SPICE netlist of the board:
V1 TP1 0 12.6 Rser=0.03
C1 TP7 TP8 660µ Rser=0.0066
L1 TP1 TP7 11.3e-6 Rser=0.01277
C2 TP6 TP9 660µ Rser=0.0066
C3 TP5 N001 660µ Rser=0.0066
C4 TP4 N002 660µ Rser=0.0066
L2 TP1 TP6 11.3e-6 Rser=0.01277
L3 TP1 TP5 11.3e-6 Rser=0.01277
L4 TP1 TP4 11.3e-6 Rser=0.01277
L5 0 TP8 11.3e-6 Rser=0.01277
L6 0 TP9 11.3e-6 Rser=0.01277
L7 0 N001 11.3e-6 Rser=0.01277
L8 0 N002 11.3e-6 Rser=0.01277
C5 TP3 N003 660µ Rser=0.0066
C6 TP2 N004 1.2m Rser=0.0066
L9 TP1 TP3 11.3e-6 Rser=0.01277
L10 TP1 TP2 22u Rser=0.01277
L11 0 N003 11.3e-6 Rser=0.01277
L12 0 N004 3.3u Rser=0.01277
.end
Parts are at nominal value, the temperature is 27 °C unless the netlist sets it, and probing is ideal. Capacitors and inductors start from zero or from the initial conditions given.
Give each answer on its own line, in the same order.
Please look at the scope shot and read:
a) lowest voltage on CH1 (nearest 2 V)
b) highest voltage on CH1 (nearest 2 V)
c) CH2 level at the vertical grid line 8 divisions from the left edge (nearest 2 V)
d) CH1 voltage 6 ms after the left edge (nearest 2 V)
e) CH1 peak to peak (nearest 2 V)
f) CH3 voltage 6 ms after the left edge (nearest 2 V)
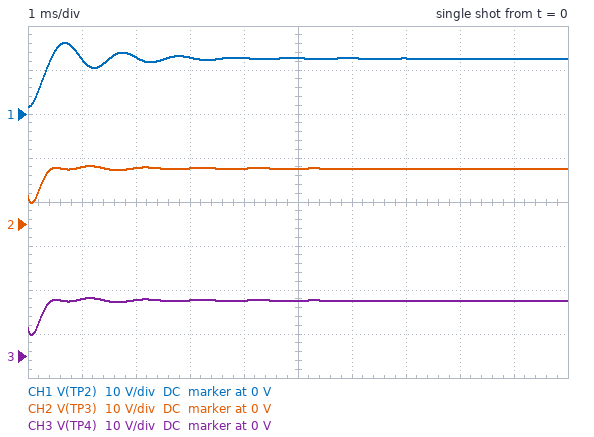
2 V
16 V
12 V
12 V
14 V
12 V
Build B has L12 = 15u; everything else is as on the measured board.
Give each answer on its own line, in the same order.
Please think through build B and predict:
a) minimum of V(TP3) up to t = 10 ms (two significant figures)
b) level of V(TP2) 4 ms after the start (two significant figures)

4.9 V
12 V
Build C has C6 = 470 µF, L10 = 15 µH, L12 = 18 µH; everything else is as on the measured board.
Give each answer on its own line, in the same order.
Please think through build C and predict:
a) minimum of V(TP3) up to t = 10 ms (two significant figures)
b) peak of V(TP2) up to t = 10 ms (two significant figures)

4.9 V
14 V
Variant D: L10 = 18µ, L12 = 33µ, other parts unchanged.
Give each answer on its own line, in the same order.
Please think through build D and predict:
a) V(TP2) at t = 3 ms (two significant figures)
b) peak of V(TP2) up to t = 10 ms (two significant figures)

12 V
15 V
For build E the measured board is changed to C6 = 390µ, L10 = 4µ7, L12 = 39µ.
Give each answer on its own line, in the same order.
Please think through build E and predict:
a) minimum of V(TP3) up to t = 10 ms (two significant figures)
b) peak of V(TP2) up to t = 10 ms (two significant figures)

4.9 V
14 V
